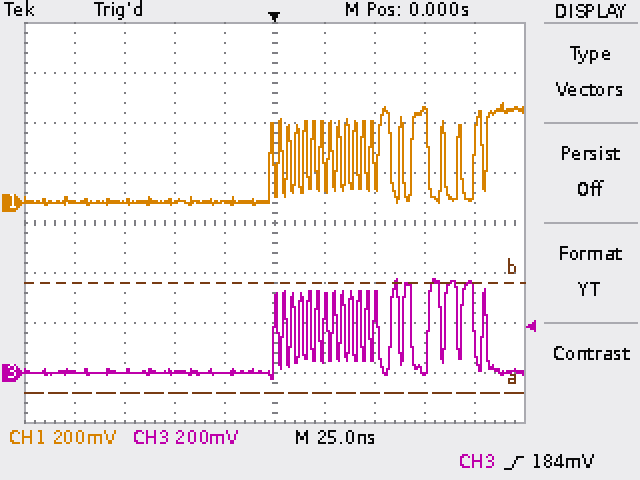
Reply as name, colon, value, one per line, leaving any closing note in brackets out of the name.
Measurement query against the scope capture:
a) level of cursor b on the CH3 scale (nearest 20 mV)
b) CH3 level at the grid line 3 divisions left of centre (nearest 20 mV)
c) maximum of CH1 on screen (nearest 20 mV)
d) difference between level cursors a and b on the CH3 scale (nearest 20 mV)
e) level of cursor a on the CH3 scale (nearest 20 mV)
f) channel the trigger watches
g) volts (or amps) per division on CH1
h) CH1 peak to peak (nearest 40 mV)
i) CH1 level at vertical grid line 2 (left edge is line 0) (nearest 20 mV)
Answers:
level of cursor b on the CH3 scale: 360 mV
CH3 level at the grid line 3 divisions left of centre: 0 mV
maximum of CH1 on screen: 400 mV
difference between level cursors a and b on the CH3 scale: 440 mV
level of cursor a on the CH3 scale: -80 mV
channel the trigger watches: CH3
volts (or amps) per division on CH1: 200 mV
CH1 peak to peak: 400 mV
CH1 level at vertical grid line 2 (left edge is line 0): 0 mV
